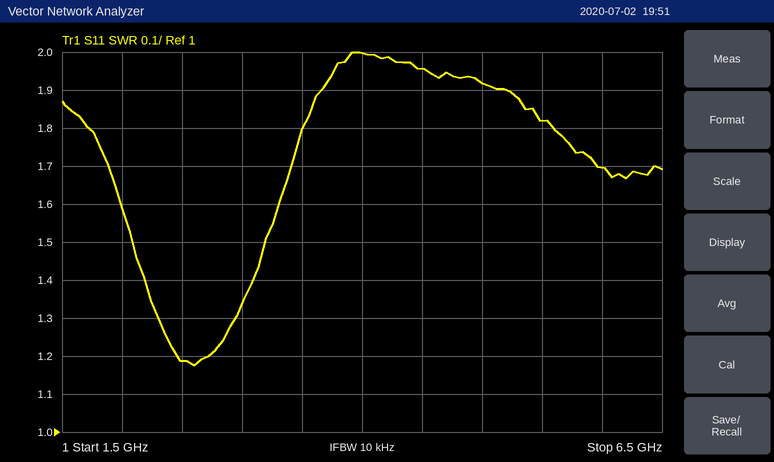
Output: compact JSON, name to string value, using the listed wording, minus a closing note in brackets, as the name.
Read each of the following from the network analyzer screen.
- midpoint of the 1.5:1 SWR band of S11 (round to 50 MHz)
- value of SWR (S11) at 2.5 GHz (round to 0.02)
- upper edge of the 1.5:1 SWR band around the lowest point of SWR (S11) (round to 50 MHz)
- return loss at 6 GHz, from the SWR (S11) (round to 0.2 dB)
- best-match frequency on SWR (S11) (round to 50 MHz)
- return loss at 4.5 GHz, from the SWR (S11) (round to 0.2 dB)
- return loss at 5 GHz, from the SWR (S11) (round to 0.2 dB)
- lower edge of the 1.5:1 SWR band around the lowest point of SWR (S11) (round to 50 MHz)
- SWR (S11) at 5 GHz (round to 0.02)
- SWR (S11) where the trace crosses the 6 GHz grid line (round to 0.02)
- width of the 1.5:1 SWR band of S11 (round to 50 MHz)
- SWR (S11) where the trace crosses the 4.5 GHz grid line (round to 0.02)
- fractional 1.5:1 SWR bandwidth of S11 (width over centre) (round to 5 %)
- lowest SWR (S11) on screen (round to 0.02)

{"midpoint of the 1.5:1 SWR band of S11": "2.65 GHz", "value of SWR (S11) at 2.5 GHz": "1.18", "upper edge of the 1.5:1 SWR band around the lowest point of SWR (S11)": "3.20 GHz", "return loss at 6 GHz, from the SWR (S11)": "11.8 dB", "best-match frequency on SWR (S11)": "2.60 GHz", "return loss at 4.5 GHz, from the SWR (S11)": "9.8 dB", "return loss at 5 GHz, from the SWR (S11)": "10.0 dB", "lower edge of the 1.5:1 SWR band around the lowest point of SWR (S11)": "2.10 GHz", "SWR (S11) at 5 GHz": "1.92", "SWR (S11) where the trace crosses the 6 GHz grid line": "1.70", "width of the 1.5:1 SWR band of S11": "1.10 GHz", "SWR (S11) where the trace crosses the 4.5 GHz grid line": "1.96", "fractional 1.5:1 SWR bandwidth of S11 (width over centre)": "40 %", "lowest SWR (S11) on screen": "1.18"}
